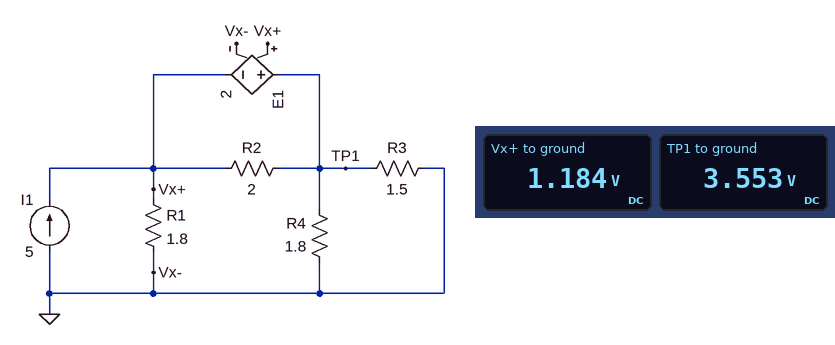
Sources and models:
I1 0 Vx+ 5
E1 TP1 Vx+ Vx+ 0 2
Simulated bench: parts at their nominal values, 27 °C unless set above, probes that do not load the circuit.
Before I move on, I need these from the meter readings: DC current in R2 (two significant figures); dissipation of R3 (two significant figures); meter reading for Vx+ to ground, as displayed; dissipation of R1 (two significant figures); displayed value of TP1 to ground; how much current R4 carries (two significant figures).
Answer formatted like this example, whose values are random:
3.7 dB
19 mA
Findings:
1.2 A
8.4 W
1.184 V
780 mW
3.553 V
2.0 A
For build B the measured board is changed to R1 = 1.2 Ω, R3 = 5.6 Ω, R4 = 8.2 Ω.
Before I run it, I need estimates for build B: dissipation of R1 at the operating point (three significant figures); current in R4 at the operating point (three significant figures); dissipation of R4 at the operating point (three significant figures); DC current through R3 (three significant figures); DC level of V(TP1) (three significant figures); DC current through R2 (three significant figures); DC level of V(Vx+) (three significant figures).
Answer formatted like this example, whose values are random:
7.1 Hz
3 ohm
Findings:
6.92 W
1.05 A
9.12 W
1.54 A
8.65 V
2.88 A
2.88 V
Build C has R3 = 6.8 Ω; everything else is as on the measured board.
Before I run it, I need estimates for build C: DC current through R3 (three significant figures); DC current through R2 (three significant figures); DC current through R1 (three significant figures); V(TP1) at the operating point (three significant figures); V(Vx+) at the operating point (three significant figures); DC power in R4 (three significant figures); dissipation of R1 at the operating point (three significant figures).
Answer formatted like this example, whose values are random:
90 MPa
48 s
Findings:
828 mA
1.88 A
1.04 A
5.63 V
1.88 V
17.6 W
1.96 W
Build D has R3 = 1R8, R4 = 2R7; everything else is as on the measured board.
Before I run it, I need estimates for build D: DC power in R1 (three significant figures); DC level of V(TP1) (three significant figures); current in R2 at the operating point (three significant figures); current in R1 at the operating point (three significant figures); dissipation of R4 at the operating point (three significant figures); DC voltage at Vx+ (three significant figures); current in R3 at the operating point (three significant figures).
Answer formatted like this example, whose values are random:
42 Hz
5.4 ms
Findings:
1.25 W
4.50 V
1.50 A
833 mA
7.50 W
1.50 V
2.50 A
